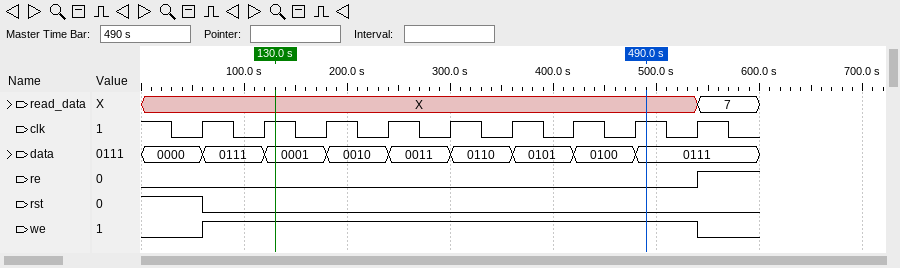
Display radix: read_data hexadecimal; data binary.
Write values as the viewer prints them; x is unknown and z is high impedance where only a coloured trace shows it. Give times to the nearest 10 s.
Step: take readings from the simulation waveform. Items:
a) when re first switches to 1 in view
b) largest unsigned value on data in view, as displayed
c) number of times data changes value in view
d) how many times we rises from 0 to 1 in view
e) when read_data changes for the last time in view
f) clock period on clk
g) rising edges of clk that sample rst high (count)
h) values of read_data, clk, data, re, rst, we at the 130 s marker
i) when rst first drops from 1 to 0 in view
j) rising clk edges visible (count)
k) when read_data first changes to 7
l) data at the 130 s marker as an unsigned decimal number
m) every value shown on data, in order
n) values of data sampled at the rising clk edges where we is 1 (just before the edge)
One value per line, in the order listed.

540 s
0111
8
1
540 s
60 s
1
read_data=X, clk=1, data=0001, re=0, rst=0, we=1
60 s
9
540 s
1
0000, 0111, 0001, 0010, 0011, 0110, 0101, 0100, 0111
0111, 0001, 0010, 0011, 0110, 0101, 0100, 0111
